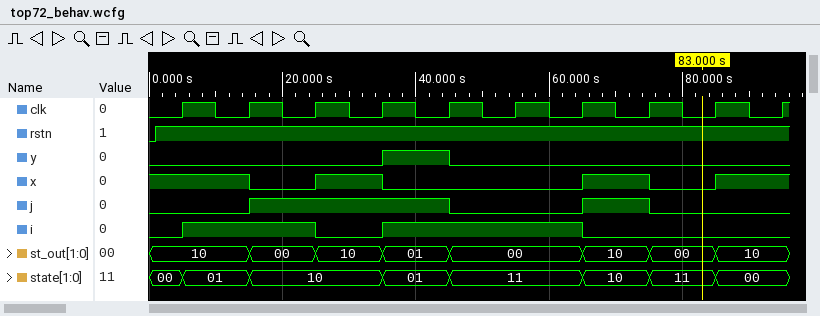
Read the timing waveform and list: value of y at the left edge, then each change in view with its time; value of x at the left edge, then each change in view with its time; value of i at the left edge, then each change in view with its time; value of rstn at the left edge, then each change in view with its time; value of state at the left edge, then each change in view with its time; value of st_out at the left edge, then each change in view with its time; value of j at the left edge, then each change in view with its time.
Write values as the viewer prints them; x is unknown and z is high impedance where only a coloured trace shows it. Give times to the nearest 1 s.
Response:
0, 1 at 35 s, 0 at 45 s
1, 0 at 15 s, 1 at 25 s, 0 at 35 s, 1 at 65 s, 0 at 75 s, 1 at 85 s
0, 1 at 5 s, 0 at 25 s, 1 at 35 s, 0 at 65 s
0, 1 at 1 s
00, 01 at 5 s, 10 at 15 s, 01 at 35 s, 11 at 45 s, 10 at 65 s, 11 at 75 s, 00 at 85 s
10, 00 at 15 s, 10 at 25 s, 01 at 35 s, 00 at 45 s, 10 at 65 s, 00 at 75 s, 10 at 85 s
0, 1 at 15 s, 0 at 45 s, 1 at 65 s, 0 at 75 s
